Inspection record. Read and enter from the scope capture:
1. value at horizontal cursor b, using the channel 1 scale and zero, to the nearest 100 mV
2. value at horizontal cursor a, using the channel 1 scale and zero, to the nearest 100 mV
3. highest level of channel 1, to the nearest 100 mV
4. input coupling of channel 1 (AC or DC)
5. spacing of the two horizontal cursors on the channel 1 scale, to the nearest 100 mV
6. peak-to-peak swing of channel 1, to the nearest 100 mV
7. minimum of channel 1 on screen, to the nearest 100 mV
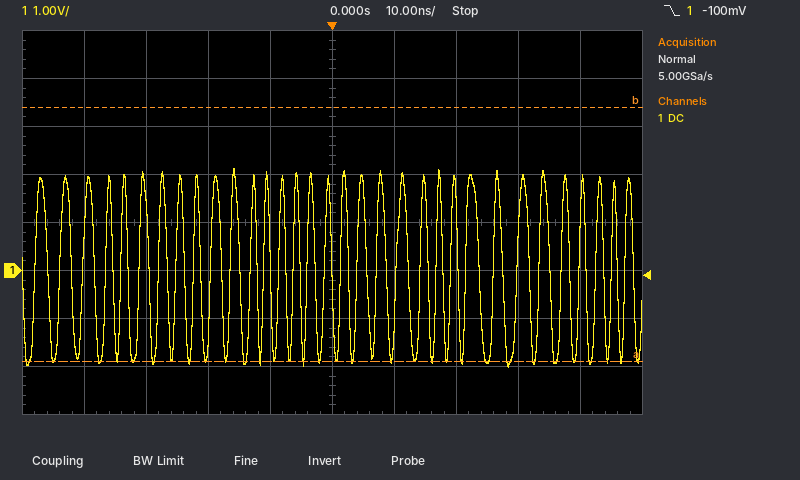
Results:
3.4 V
-1.9 V
2.1 V
DC
5.3 V
4.1 V
-2.0 V
